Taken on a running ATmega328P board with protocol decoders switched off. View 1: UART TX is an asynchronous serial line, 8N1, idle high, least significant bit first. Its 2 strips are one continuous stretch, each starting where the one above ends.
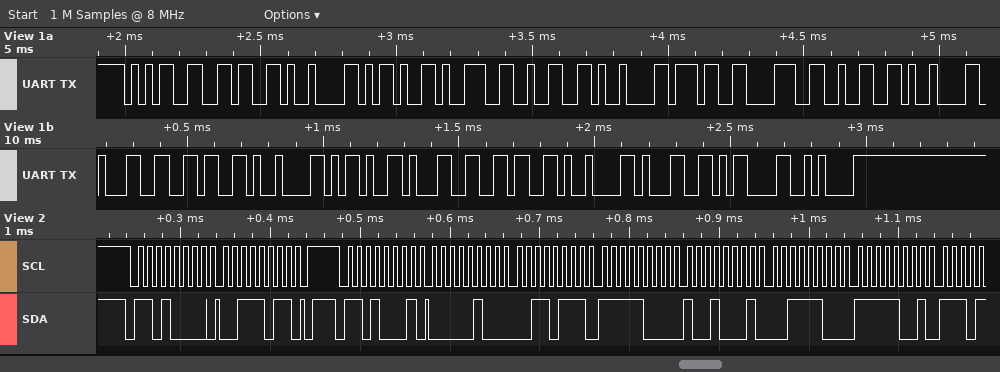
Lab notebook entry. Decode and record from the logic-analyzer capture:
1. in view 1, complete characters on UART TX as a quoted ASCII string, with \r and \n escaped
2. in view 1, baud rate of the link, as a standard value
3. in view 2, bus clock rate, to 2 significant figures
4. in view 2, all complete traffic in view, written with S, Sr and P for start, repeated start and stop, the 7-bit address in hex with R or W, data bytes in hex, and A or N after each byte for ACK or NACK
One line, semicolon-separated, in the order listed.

"56\t-92\t782\t16\t-16\t1\r\n"; 38400 baud; 100 kHz; S 68W A 3B A P S 68R A 04 A 37 A F8 A 91 A 3C A F9 A
